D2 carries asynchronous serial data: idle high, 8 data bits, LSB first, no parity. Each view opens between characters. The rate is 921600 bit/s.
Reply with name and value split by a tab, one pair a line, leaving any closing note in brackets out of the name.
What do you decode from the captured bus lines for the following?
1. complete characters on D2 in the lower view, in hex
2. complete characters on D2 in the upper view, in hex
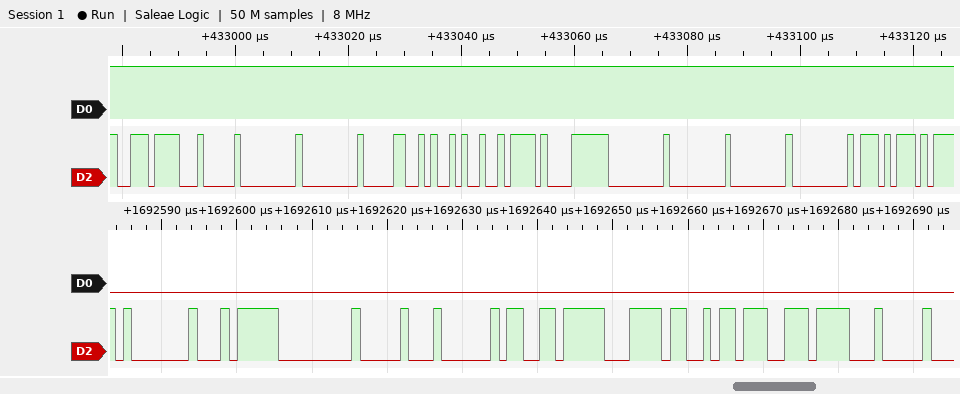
complete characters on D2 in the lower view, in hex	01, F4, 00, 10, A0, F6, BC, DA, EE, 04
complete characters on D2 in the upper view, in hex	EE, 04, 00, 00, 30, 29, 7A, F8, 00, 00, 00, 00, D7
